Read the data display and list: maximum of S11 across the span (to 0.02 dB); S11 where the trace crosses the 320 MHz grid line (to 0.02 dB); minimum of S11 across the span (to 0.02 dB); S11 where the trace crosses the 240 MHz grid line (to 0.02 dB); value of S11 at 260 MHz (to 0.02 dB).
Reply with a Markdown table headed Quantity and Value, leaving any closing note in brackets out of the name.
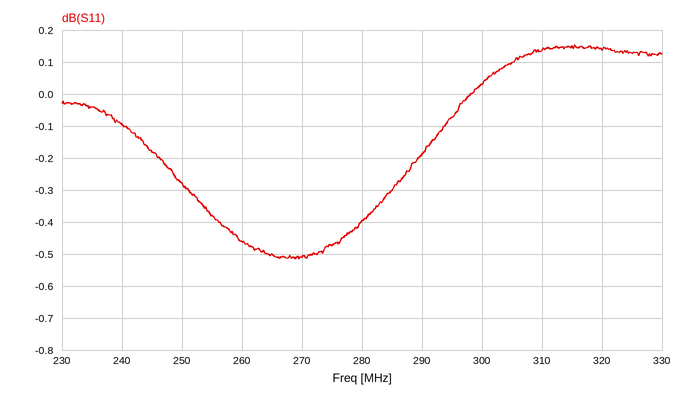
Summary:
| Quantity | Value |
|---|---|
| maximum of S11 across the span | 0.16 dB |
| S11 where the trace crosses the 320 MHz grid line | 0.14 dB |
| minimum of S11 across the span | -0.52 dB |
| S11 where the trace crosses the 240 MHz grid line | -0.10 dB |
| value of S11 at 260 MHz | -0.46 dB |
